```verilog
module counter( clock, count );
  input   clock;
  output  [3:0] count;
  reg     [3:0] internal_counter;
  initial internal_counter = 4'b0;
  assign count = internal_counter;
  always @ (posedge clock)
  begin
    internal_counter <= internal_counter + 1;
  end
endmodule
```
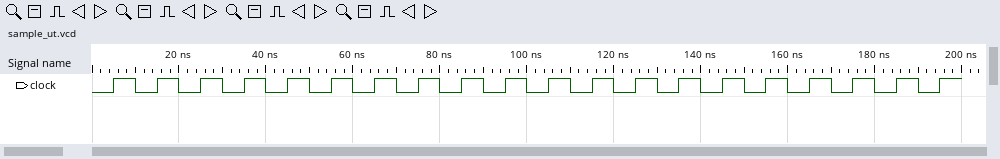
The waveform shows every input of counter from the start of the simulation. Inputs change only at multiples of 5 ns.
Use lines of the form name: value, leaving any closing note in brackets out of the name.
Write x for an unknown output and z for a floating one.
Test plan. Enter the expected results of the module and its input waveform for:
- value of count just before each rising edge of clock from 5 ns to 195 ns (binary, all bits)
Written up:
value of count just before each rising edge of clock from 5 ns to 195 ns: 0000, 0001, 0010, 0011, 0100, 0101, 0110, 0111, 1000, 1001, 1010, 1011, 1100, 1101, 1110, 1111, 0000, 0001, 0010, 0011
